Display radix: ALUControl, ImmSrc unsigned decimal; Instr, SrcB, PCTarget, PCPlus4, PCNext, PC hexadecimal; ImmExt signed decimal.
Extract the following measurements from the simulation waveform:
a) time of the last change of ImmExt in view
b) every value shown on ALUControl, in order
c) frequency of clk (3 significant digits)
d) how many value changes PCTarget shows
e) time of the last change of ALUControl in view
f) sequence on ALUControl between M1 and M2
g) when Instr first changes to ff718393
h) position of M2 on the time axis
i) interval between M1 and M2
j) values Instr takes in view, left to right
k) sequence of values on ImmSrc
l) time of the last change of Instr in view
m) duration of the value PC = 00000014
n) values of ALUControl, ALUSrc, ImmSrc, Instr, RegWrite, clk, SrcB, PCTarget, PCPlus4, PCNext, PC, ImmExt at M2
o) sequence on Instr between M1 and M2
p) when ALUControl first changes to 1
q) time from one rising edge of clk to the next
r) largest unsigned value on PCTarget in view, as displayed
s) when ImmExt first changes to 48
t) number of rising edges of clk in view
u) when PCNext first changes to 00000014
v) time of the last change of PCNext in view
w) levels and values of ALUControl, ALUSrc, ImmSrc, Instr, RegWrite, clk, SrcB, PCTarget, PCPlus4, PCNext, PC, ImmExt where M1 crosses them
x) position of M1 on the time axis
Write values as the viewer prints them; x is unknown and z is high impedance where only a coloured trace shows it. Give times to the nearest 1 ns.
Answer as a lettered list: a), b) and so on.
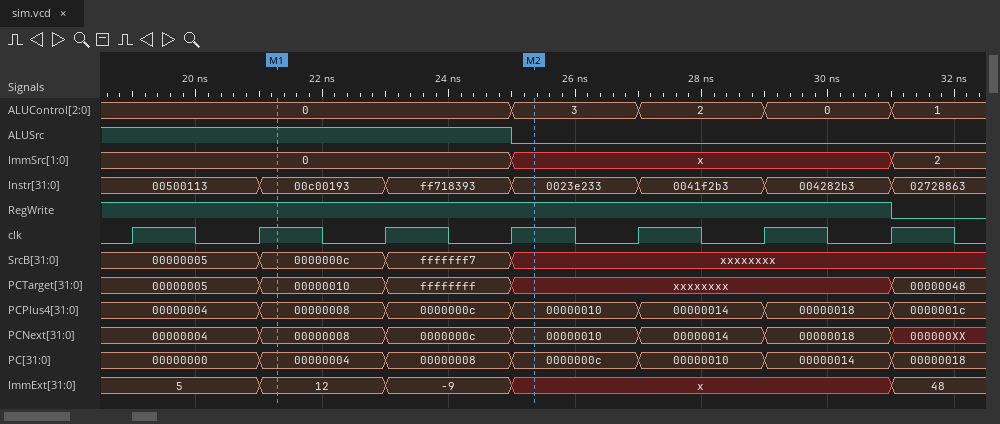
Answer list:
a) 31 ns
b) 0, 3, 2, 0, 1
c) 500 MHz
d) 4
e) 31 ns
f) 0, 3
g) 23 ns
h) 25 ns
i) 4 ns
j) 00500113, 00c00193, ff718393, 0023e233, 0041f2b3, 004282b3, 02728863
k) 0, x, 2
l) 31 ns
m) 2 ns
n) ALUControl=3, ALUSrc=0, ImmSrc=x, Instr=0023e233, RegWrite=1, clk=1, SrcB=xxxxxxxx, PCTarget=xxxxxxxx, PCPlus4=00000010, PCNext=00000010, PC=0000000c, ImmExt=x
o) 00c00193, ff718393, 0023e233
p) 31 ns
q) 2 ns
r) ffffffff
s) 31 ns
t) 7
u) 27 ns
v) 31 ns
w) ALUControl=0, ALUSrc=1, ImmSrc=0, Instr=00c00193, RegWrite=1, clk=1, SrcB=0000000c, PCTarget=00000010, PCPlus4=00000008, PCNext=00000008, PC=00000004, ImmExt=12
x) 21 ns
